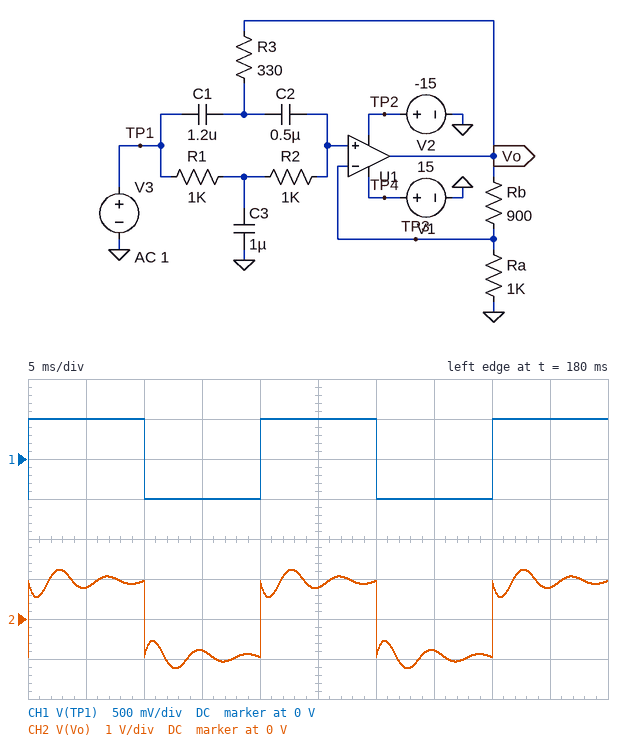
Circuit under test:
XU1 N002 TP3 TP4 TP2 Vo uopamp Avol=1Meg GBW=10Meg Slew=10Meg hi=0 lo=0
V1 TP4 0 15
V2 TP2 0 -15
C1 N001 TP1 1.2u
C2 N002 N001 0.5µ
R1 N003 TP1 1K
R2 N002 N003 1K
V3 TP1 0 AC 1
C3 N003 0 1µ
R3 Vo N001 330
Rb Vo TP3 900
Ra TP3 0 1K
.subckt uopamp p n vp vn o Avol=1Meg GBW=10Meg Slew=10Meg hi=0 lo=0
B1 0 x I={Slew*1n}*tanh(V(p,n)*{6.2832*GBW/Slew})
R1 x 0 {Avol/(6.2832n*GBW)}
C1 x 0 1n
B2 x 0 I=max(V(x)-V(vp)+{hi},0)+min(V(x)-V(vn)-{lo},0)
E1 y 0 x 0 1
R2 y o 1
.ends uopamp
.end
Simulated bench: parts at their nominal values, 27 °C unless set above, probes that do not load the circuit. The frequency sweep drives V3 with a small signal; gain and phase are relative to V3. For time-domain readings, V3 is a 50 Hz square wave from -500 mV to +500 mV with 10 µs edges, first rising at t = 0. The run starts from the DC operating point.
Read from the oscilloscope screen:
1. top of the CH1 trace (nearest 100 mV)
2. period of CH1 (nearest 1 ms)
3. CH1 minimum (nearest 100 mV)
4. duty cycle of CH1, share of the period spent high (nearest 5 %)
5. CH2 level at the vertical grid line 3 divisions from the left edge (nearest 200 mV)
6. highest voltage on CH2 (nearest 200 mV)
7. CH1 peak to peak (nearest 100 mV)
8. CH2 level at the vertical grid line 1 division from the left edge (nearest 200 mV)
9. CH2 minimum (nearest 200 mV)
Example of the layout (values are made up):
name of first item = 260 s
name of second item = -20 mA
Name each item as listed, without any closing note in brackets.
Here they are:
top of the CH1 trace = 500 mV
period of CH1 = 20 ms
CH1 minimum = -500 mV
duty cycle of CH1, share of the period spent high = 50 %
CH2 level at the vertical grid line 3 divisions from the left edge = -800 mV
highest voltage on CH2 = 1.2 V
CH1 peak to peak = 1.0 V
CH2 level at the vertical grid line 1 division from the left edge = 800 mV
CH2 minimum = -1.2 V
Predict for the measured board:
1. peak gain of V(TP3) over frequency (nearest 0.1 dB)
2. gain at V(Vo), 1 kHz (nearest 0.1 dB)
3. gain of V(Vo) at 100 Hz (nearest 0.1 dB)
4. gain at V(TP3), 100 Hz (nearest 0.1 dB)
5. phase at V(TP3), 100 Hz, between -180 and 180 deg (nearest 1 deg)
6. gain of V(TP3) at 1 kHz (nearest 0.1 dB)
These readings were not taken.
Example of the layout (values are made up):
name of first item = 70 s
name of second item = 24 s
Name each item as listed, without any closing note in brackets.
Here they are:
peak gain of V(TP3) over frequency = 0.4 dB
gain at V(Vo), 1 kHz = 5.4 dB
gain of V(Vo) at 100 Hz = 5.7 dB
gain at V(TP3), 100 Hz = 0.2 dB
phase at V(TP3), 100 Hz, between -180 and 180 deg = -5 deg
gain of V(TP3) at 1 kHz = -0.2 dB
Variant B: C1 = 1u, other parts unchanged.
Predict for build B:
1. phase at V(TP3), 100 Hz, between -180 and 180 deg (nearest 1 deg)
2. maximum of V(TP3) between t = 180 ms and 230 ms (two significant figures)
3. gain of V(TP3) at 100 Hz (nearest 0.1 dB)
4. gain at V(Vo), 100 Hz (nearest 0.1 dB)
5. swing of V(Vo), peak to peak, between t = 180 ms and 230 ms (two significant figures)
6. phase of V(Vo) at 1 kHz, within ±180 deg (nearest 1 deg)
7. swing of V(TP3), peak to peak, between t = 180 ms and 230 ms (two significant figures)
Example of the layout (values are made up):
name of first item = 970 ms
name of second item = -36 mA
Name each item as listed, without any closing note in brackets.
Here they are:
phase at V(TP3), 100 Hz, between -180 and 180 deg = -4 deg
maximum of V(TP3) between t = 180 ms and 230 ms = 610 mV
gain of V(TP3) at 100 Hz = 0 dB
gain at V(Vo), 100 Hz = 5.5 dB
swing of V(Vo), peak to peak, between t = 180 ms and 230 ms = 2.3 V
phase of V(Vo) at 1 kHz, within ±180 deg = 3 deg
swing of V(TP3), peak to peak, between t = 180 ms and 230 ms = 1.2 V
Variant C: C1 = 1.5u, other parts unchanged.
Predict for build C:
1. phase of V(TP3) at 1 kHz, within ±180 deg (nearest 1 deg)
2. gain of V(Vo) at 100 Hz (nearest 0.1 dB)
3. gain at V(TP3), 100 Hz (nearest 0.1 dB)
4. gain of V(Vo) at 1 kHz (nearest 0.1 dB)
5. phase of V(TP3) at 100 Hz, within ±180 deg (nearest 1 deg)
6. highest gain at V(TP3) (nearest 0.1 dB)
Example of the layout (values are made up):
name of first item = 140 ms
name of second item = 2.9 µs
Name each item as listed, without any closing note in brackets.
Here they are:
phase of V(TP3) at 1 kHz, within ±180 deg = 7 deg
gain of V(Vo) at 100 Hz = 6.0 dB
gain at V(TP3), 100 Hz = 0.5 dB
gain of V(Vo) at 1 kHz = 5.2 dB
phase of V(TP3) at 100 Hz, within ±180 deg = -6 deg
highest gain at V(TP3) = 0.9 dB
